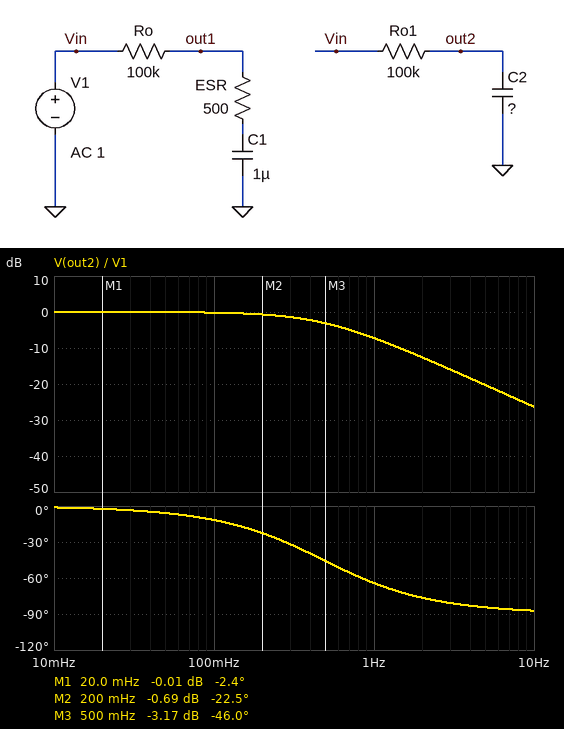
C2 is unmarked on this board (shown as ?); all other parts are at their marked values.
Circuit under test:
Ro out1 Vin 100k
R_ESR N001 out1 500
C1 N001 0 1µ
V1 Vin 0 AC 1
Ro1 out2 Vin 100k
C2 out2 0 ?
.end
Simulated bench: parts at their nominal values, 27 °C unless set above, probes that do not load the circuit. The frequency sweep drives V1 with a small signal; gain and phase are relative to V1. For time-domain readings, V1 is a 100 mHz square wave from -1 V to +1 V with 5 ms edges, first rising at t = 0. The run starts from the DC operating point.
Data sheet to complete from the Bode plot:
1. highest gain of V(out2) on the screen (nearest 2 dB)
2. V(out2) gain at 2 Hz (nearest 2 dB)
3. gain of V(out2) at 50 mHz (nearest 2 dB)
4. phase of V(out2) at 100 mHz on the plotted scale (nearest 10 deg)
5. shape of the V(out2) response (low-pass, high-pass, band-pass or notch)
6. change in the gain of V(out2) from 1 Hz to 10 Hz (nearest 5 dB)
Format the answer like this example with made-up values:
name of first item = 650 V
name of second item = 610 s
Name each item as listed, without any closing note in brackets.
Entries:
highest gain of V(out2) on the screen = 0 dB
V(out2) gain at 2 Hz = -12 dB
gain of V(out2) at 50 mHz = 0 dB
phase of V(out2) at 100 mHz on the plotted scale = -10 deg
shape of the V(out2) response = low-pass
change in the gain of V(out2) from 1 Hz to 10 Hz = -20 dB
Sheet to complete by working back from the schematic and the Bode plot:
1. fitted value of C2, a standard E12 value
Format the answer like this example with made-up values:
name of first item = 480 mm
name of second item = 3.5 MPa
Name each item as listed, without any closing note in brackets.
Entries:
fitted value of C2, a standard E12 value = 3.3 µF
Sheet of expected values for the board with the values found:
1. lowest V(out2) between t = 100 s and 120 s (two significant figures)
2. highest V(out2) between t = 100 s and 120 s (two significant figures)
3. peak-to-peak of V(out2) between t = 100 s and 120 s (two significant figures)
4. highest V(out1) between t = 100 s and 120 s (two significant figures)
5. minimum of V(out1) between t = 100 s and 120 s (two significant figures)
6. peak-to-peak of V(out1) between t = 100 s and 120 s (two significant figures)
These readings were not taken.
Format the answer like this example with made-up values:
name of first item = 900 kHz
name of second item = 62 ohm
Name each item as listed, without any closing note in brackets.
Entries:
lowest V(out2) between t = 100 s and 120 s = -1.0 V
highest V(out2) between t = 100 s and 120 s = 1.0 V
peak-to-peak of V(out2) between t = 100 s and 120 s = 2.0 V
highest V(out1) between t = 100 s and 120 s = 1.0 V
minimum of V(out1) between t = 100 s and 120 s = -1.0 V
peak-to-peak of V(out1) between t = 100 s and 120 s = 2.0 V
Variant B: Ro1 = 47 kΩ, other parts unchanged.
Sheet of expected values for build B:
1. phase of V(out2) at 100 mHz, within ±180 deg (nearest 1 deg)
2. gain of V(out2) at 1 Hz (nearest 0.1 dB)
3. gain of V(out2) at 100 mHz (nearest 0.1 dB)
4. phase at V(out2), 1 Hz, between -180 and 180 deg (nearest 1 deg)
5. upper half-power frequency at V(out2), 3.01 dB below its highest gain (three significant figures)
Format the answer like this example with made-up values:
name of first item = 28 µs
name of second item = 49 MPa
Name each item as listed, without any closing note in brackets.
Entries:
phase of V(out2) at 100 mHz, within ±180 deg = -6 deg
gain of V(out2) at 1 Hz = -2.9 dB
gain of V(out2) at 100 mHz = 0 dB
phase at V(out2), 1 Hz, between -180 and 180 deg = -44 deg
upper half-power frequency at V(out2), 3.01 dB below its highest gain = 1.03 Hz
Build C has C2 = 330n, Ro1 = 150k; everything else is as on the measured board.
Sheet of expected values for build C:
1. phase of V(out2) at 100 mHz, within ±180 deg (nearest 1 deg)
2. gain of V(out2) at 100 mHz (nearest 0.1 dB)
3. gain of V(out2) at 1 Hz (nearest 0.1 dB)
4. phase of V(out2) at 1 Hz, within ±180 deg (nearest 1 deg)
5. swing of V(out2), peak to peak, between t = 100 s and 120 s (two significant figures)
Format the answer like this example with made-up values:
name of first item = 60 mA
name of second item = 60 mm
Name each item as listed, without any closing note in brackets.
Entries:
phase of V(out2) at 100 mHz, within ±180 deg = -2 deg
gain of V(out2) at 100 mHz = 0 dB
gain of V(out2) at 1 Hz = -0.4 dB
phase of V(out2) at 1 Hz, within ±180 deg = -17 deg
swing of V(out2), peak to peak, between t = 100 s and 120 s = 2.0 V
